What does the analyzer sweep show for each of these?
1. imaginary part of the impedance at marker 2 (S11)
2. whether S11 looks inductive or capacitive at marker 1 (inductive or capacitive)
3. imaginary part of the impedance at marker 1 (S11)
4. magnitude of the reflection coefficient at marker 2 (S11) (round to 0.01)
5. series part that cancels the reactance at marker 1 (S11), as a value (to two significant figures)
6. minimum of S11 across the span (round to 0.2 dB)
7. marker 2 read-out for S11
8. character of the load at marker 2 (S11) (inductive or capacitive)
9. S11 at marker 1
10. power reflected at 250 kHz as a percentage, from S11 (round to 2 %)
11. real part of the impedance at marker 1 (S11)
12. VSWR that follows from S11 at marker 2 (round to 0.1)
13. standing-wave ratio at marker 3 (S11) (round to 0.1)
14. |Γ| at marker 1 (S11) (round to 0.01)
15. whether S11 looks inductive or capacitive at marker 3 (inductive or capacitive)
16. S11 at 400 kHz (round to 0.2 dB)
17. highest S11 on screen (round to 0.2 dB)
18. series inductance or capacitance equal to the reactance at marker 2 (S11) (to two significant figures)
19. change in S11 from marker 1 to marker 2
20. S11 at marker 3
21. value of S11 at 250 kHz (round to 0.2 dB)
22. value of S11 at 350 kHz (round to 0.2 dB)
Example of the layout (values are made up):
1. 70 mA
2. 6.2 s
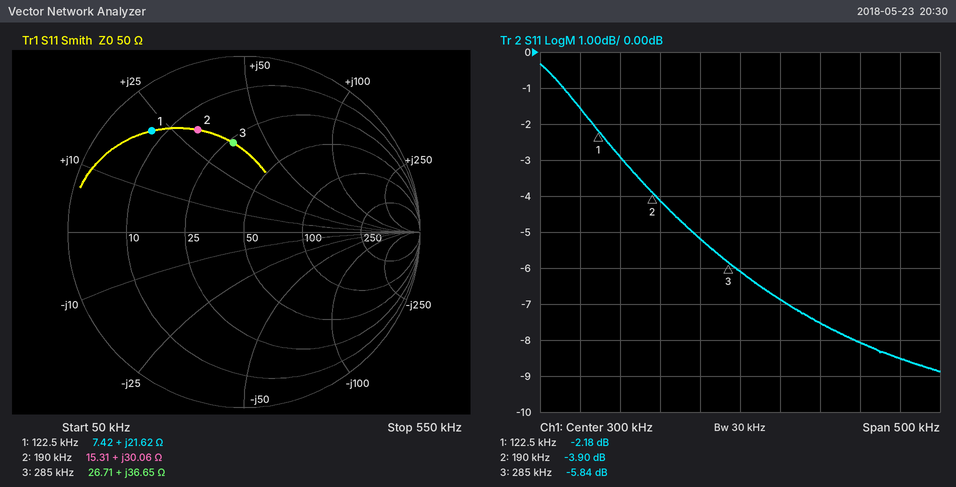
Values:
1. +30.06 Ω
2. inductive
3. +21.62 Ω
4. 0.64
5. 60 nF
6. -8.8 dB
7. -3.90 dB
8. inductive
9. -2.18 dB
10. 30 %
11. 7.42 Ω
12. 4.5
13. 3.1
14. 0.78
15. inductive
16. -7.6 dB
17. -0.4 dB
18. 25 µH
19. -1.72 dB
20. -5.84 dB
21. -5.2 dB
22. -6.8 dB
